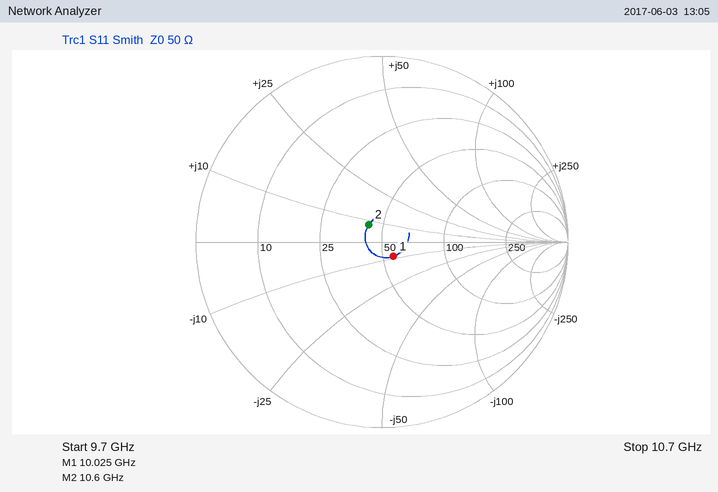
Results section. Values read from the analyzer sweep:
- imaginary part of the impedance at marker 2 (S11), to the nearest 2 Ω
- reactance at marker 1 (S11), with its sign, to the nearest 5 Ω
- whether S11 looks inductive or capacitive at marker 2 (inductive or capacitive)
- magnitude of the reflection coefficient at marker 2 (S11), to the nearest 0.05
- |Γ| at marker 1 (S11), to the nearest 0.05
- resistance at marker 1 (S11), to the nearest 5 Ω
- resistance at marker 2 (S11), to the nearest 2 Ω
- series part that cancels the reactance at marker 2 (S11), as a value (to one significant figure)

+8 Ω
-10 Ω
inductive
0.10
0.10
55 Ω
42 Ω
2 pF
